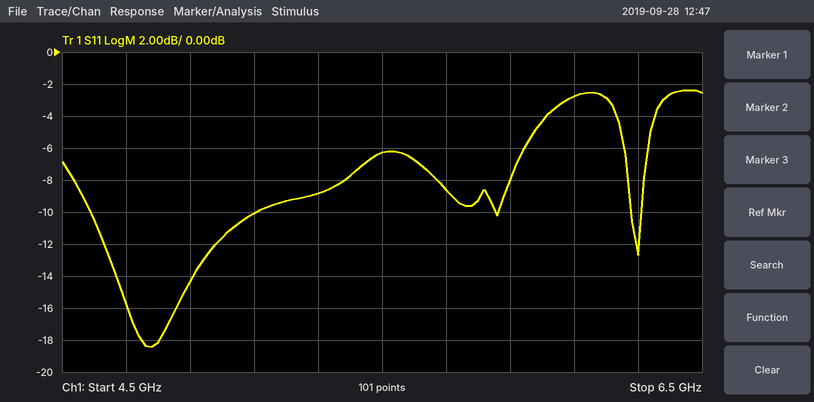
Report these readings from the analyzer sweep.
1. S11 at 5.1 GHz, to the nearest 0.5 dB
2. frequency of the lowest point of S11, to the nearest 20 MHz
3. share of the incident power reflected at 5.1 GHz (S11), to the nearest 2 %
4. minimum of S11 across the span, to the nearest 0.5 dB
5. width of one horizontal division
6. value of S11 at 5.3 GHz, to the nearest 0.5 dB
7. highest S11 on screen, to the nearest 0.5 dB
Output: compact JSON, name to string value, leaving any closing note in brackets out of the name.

{"S11 at 5.1 GHz, to the nearest 0.5 dB": "-10.0 dB", "frequency of the lowest point of S11, to the nearest 20 MHz": "4.78 GHz", "share of the incident power reflected at 5.1 GHz (S11), to the nearest 2 %": "10 %", "minimum of S11 across the span, to the nearest 0.5 dB": "-18.5 dB", "width of one horizontal division": "200 MHz", "value of S11 at 5.3 GHz, to the nearest 0.5 dB": "-9.0 dB", "highest S11 on screen, to the nearest 0.5 dB": "-2.5 dB"}
